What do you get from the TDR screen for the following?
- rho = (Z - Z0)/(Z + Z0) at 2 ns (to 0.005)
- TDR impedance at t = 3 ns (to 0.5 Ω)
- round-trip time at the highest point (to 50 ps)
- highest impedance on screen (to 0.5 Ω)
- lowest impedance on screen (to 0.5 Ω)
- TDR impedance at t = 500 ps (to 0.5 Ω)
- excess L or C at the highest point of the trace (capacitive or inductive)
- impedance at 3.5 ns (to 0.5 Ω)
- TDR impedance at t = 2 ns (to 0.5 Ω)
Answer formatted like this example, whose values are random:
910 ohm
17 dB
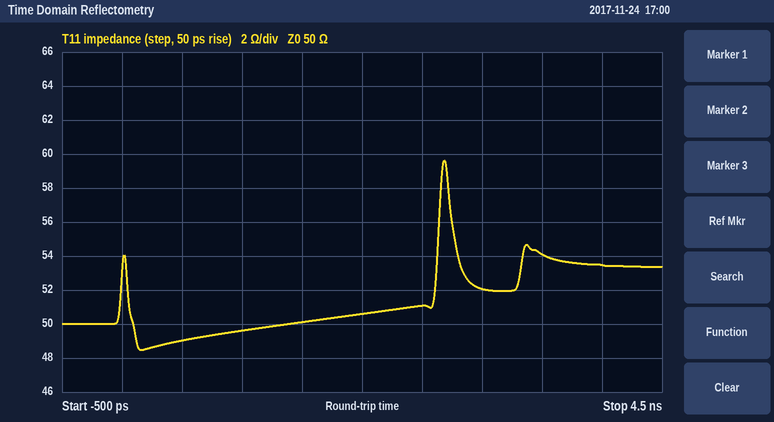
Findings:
+0.005
52.0 Ω
2.70 ns
59.5 Ω
48.5 Ω
49.0 Ω
inductive
54.0 Ω
50.5 Ω
